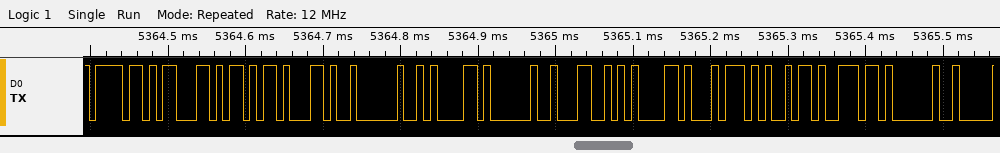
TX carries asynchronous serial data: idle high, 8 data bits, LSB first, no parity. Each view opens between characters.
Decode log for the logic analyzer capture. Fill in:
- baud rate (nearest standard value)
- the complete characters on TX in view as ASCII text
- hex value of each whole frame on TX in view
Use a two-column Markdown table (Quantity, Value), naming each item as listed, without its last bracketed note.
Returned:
| Quantity | Value |
|---|---|
| baud rate | 115200 baud |
| the complete characters on TX in view as ASCII text | "ock, a Latin " |
| hex value of each whole frame on TX in view | 6F, 63, 6B, 2C, 20, 61, 20, 4C, 61, 74, 69, 6E, 20 |
